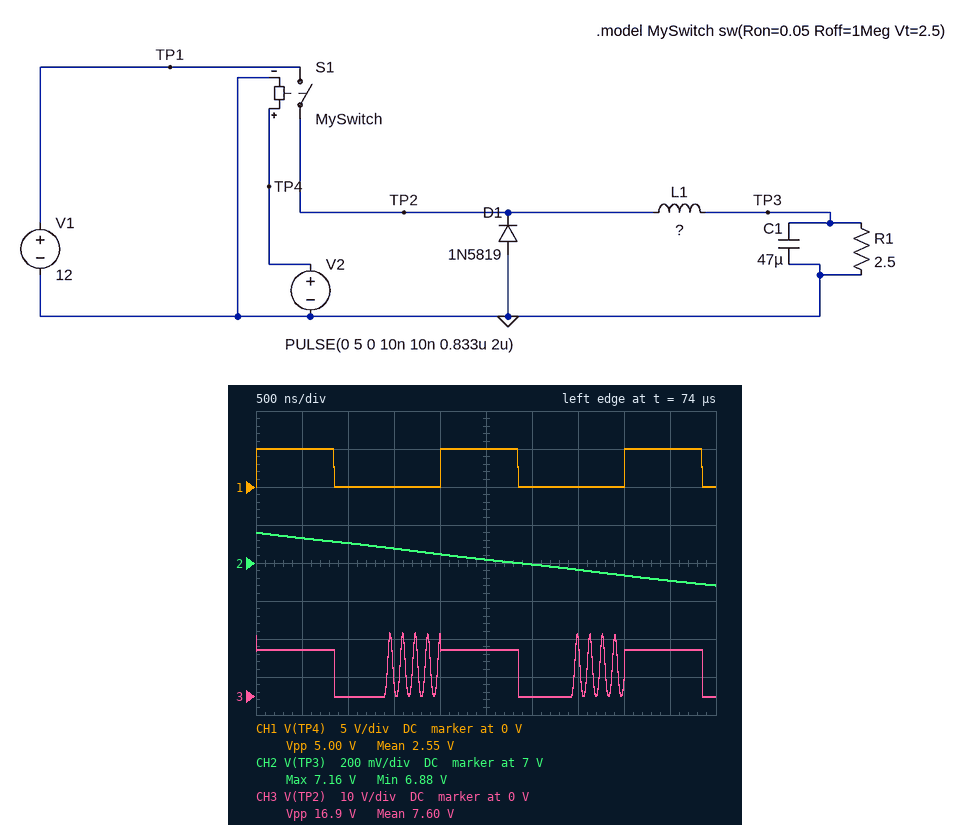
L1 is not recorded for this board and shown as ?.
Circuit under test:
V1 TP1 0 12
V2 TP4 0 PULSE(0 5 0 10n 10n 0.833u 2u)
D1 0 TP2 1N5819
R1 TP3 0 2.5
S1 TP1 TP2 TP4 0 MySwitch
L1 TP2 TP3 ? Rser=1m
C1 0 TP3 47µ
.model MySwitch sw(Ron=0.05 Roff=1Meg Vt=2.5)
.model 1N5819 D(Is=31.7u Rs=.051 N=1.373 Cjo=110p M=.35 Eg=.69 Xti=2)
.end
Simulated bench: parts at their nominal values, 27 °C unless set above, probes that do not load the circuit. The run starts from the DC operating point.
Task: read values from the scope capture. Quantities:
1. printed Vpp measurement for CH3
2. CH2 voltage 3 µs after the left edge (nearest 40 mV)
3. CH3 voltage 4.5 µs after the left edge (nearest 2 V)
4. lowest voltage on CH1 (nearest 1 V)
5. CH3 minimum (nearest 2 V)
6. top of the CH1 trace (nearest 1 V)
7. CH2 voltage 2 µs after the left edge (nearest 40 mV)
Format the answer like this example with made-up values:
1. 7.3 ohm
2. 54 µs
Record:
1. 16.9 V
2. 7.00 V
3. 12 V
4. 0 V
5. 0 V
6. 5 V
7. 7.04 V
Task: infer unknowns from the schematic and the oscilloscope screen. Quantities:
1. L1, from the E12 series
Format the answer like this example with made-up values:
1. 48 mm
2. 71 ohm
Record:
1. 8.2 µH
